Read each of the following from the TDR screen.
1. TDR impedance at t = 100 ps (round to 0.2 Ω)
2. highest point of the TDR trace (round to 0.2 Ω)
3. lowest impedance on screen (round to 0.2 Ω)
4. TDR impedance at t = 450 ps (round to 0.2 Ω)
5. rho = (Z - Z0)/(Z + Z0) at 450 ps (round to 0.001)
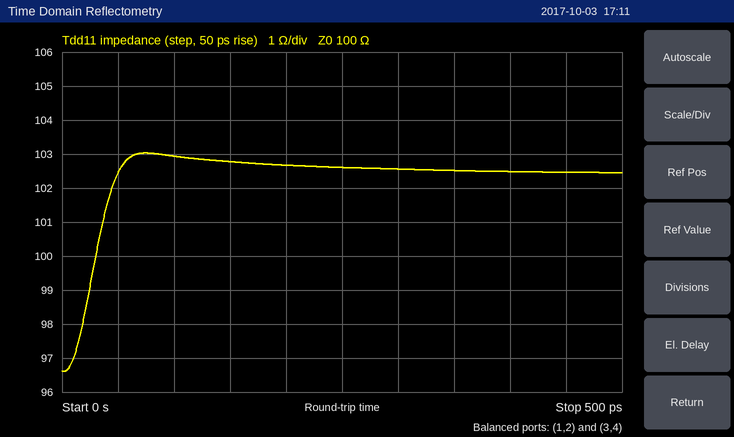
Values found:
103.0 Ω
103.0 Ω
96.6 Ω
102.4 Ω
+0.012
